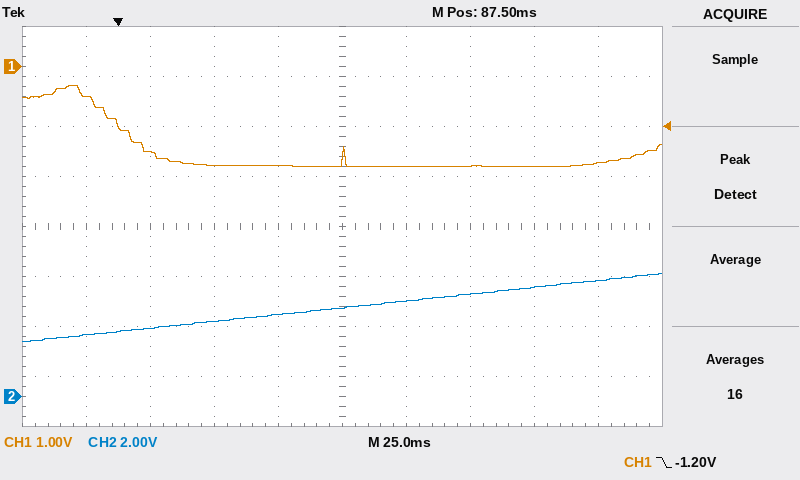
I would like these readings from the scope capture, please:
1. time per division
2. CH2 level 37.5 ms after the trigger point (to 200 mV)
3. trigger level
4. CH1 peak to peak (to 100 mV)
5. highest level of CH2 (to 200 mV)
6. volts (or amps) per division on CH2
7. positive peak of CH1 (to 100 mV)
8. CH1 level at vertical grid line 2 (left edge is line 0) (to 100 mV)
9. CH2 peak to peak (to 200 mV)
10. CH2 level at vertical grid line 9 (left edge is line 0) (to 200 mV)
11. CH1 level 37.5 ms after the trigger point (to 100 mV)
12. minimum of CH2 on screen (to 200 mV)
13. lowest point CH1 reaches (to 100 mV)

25 ms
3.0 V
-1.20 V
1.6 V
5.0 V
2 V
-400 mV
-1.7 V
2.8 V
4.6 V
-2.0 V
2.2 V
-2.0 V
